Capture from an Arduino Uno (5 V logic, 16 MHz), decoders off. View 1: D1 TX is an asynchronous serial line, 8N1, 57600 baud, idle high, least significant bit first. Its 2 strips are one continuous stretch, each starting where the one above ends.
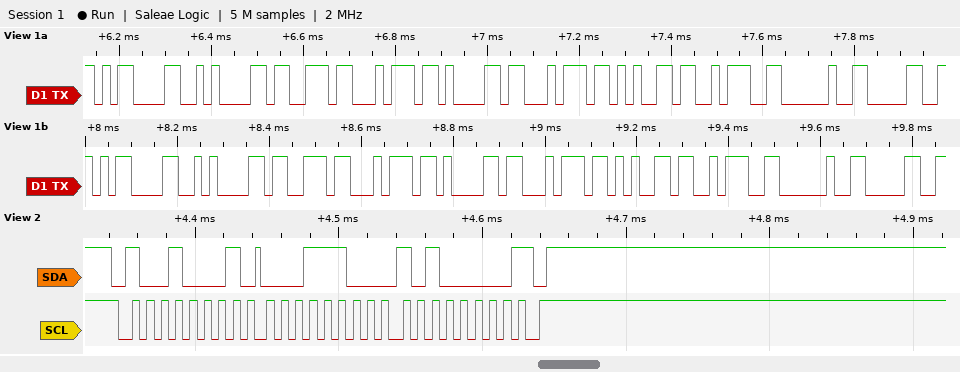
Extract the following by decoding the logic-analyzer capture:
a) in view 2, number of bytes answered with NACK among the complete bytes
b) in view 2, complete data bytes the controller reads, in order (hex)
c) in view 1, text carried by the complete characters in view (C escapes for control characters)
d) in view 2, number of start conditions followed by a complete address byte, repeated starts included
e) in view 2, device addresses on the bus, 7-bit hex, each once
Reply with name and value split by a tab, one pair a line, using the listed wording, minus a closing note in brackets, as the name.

in view 2, number of bytes answered with NACK among the complete bytes	1
in view 2, complete data bytes the controller reads, in order	1C A0
in view 1, text carried by the complete characters in view	"\r\nstate: 0\r\nstate: 0"
in view 2, number of start conditions followed by a complete address byte, repeated starts included	1
in view 2, device addresses on the bus, 7-bit hex, each once	0x48
